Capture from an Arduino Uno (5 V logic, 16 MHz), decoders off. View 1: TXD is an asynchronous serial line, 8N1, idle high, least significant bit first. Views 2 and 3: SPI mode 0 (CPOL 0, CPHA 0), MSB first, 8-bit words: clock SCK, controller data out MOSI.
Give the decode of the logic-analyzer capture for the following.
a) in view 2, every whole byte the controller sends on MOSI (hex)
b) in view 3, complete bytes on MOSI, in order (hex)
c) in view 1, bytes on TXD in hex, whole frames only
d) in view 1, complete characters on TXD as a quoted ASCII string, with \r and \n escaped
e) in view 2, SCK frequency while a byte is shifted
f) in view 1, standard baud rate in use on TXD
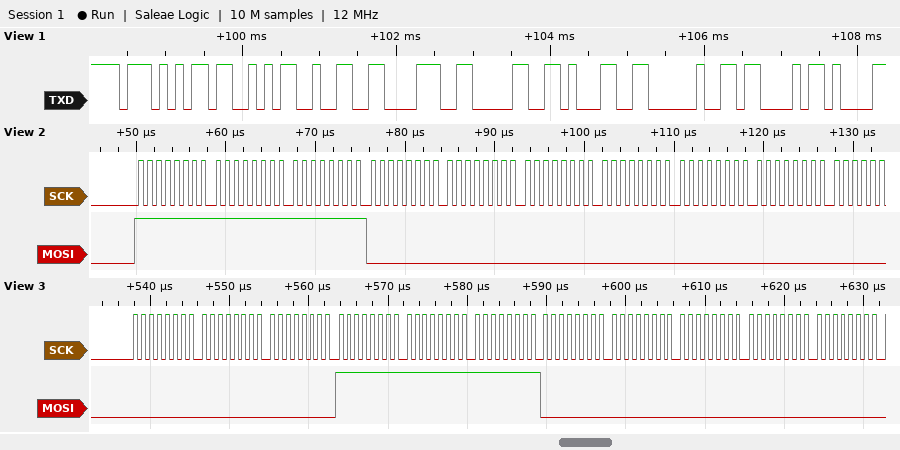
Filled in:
FF FF FF 00 00 00 00 00 00
00 00 00 FF FF FF 00 00 00 00 00
57 53 32 38 30 31 20 43
"WS2801 C"
1 MHz
9600 baud
